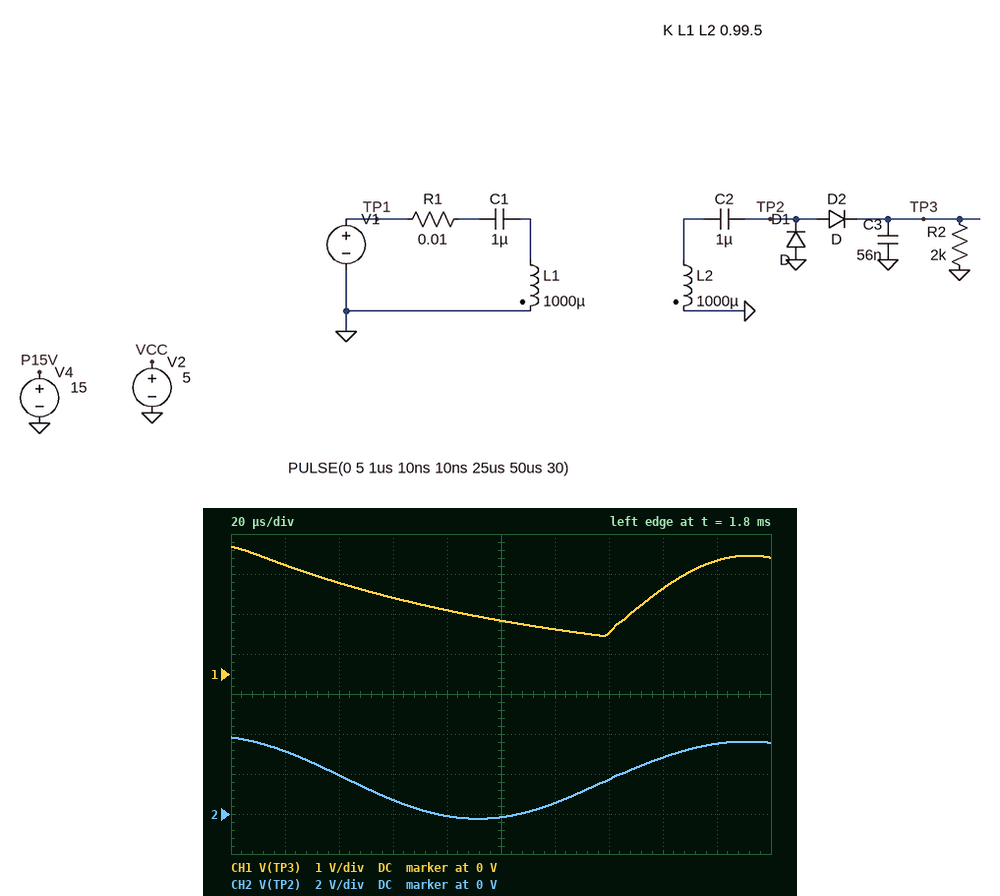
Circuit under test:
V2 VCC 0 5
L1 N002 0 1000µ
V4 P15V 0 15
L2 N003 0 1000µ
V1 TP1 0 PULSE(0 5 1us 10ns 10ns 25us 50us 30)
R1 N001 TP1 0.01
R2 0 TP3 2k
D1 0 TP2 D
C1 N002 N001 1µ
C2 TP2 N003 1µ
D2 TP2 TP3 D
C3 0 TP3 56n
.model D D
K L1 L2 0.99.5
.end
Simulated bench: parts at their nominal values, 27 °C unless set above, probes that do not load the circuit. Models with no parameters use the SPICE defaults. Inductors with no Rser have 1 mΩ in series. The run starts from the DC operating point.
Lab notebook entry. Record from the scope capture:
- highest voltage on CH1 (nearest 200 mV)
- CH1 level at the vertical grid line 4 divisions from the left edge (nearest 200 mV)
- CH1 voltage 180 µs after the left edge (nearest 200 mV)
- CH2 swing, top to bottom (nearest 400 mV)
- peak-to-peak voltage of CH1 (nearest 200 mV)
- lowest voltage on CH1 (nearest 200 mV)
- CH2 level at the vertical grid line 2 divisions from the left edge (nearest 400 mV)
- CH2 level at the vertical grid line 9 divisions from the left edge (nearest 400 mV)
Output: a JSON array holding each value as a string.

["3.2 V", "1.6 V", "2.8 V", "4.0 V", "2.2 V", "1.0 V", "2.0 V", "3.6 V"]
